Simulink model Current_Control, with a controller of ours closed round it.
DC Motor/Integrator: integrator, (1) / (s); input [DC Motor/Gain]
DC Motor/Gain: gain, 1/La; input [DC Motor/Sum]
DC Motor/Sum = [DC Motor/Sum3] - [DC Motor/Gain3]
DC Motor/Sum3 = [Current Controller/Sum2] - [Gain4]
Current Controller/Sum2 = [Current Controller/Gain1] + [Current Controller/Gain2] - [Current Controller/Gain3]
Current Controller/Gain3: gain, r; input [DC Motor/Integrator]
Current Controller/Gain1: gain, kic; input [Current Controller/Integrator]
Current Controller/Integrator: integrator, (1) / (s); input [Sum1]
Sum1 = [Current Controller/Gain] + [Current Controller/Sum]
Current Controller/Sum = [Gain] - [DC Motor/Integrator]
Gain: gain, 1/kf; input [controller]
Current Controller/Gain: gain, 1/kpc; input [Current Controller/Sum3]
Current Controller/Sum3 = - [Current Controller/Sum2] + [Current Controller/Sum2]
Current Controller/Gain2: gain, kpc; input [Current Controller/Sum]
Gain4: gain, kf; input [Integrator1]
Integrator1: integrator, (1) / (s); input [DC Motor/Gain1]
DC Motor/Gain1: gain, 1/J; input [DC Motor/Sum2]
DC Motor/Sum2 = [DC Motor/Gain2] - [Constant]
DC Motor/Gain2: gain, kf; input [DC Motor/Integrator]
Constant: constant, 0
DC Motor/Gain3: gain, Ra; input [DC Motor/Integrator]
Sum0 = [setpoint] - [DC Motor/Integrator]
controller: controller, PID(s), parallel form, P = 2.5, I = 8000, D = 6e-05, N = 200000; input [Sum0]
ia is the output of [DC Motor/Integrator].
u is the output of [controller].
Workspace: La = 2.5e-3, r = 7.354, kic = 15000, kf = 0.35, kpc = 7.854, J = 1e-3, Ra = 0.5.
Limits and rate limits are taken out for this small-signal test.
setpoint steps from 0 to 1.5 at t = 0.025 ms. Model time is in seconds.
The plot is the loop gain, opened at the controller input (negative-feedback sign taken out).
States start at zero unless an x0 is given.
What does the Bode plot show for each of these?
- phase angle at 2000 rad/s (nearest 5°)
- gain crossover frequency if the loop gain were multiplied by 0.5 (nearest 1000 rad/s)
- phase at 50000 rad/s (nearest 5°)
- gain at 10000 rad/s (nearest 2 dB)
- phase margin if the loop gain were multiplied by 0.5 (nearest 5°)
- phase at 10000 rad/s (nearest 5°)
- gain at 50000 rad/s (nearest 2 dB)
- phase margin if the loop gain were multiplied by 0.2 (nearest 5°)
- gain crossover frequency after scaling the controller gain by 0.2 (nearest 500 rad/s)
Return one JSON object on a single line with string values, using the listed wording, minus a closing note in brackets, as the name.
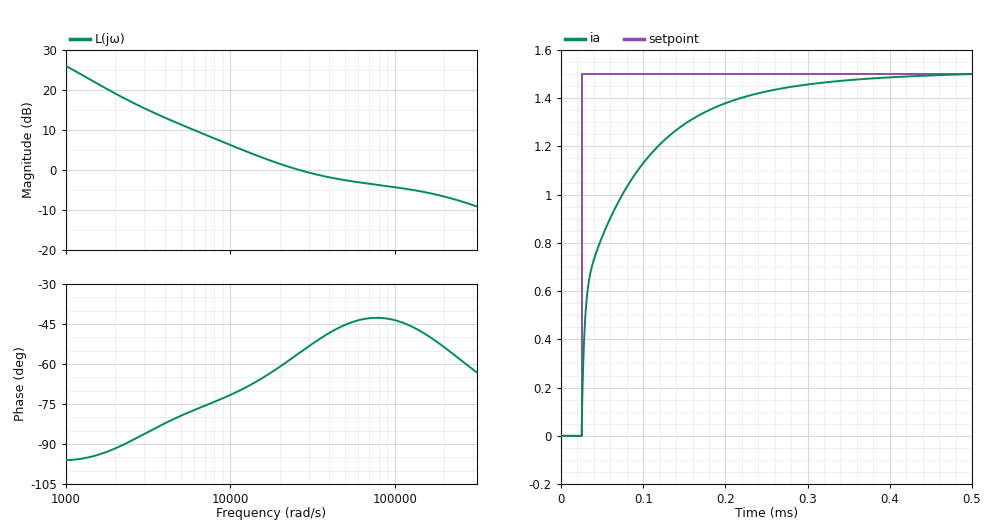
{"phase angle at 2000 rad/s": "-90°", "gain crossover frequency if the loop gain were multiplied by 0.5": "10000 rad/s", "phase at 50000 rad/s": "-45°", "gain at 10000 rad/s": "6 dB", "phase margin if the loop gain were multiplied by 0.5": "110°", "phase at 10000 rad/s": "-70°", "gain at 50000 rad/s": "-2 dB", "phase margin if the loop gain were multiplied by 0.2": "95°", "gain crossover frequency after scaling the controller gain by 0.2": "3500 rad/s"}
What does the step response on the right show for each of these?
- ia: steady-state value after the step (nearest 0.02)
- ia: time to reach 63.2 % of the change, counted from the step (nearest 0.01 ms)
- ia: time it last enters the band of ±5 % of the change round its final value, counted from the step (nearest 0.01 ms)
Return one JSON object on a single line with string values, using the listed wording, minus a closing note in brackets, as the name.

{"ia: steady-state value after the step": "1.50", "ia: time to reach 63.2 % of the change, counted from the step": "0.04 ms", "ia: time it last enters the band of ±5 % of the change round its final value, counted from the step": "0.22 ms"}
